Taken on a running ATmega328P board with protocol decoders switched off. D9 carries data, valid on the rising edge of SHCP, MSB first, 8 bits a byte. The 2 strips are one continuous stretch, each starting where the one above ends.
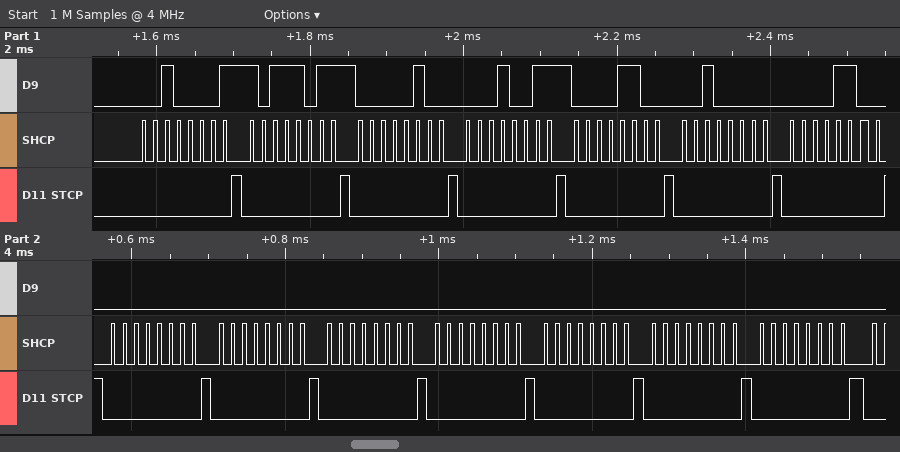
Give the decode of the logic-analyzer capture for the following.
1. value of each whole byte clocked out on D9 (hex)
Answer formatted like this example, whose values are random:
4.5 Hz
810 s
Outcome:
21 BB 04 13 0C 20 0C 00 00 00 00 00 00 00
